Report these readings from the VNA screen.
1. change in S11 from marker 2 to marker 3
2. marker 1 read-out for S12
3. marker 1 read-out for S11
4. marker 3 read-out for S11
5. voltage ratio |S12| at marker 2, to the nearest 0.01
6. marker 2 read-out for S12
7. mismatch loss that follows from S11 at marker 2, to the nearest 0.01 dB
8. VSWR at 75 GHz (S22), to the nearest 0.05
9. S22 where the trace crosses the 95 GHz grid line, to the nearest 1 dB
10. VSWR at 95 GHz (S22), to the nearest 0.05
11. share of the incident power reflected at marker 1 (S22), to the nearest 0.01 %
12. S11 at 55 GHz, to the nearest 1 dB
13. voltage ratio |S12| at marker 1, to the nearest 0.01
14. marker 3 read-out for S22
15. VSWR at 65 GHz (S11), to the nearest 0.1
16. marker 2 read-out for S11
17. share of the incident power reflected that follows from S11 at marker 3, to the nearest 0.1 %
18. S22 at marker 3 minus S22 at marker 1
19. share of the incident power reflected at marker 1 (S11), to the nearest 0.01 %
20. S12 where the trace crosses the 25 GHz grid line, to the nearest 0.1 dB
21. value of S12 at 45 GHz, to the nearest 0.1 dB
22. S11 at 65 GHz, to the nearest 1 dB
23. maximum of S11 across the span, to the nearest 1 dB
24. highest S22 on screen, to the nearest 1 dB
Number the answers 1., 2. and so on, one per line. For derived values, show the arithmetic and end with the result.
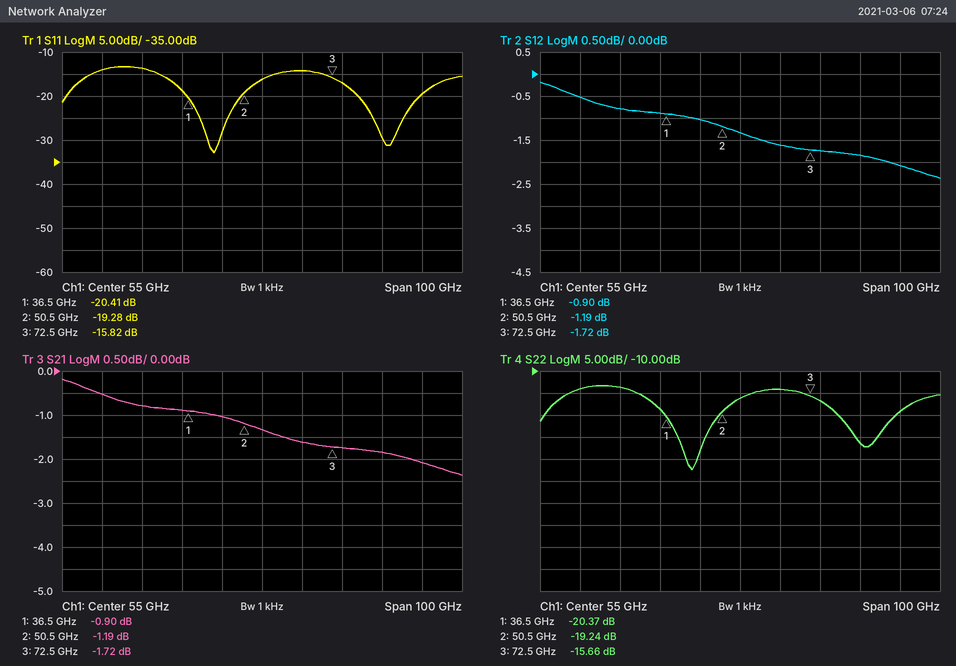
1. -15.82 − (-19.28) = 3.46 dB
2. -0.90 dB
3. -20.41 dB
4. -15.82 dB
5. 10^(-1.19/20) ≈ 0.87
6. -1.19 dB
7. −10 log10(1 − 10^(-19.28/10)) ≈ 0.05 dB
8. |Γ| = 10^(-17/20) = 0.1413; VSWR = (1 + 0.1413)/(1 − 0.1413) ≈ 1.33, so 1.35 to the nearest 0.05
9. -19 dB
10. |Γ| = 10^(-19/20) = 0.1122; VSWR = (1 + 0.1122)/(1 − 0.1122) ≈ 1.25
11. 10^(-20.37/10) ≈ 0.92 %
12. -16 dB
13. 10^(-0.9/20) ≈ 0.90
14. -15.66 dB
15. |Γ| = 10^(-14/20) = 0.1995; VSWR = (1 + 0.1995)/(1 − 0.1995) ≈ 1.5
16. -19.28 dB
17. 10^(-15.82/10) ≈ 2.6 %
18. -15.66 − (-20.37) = 4.71 dB
19. 10^(-20.41/10) ≈ 0.91 %
20. -0.8 dB
21. -1.0 dB
22. -14 dB
23. -13 dB
24. -13 dB
